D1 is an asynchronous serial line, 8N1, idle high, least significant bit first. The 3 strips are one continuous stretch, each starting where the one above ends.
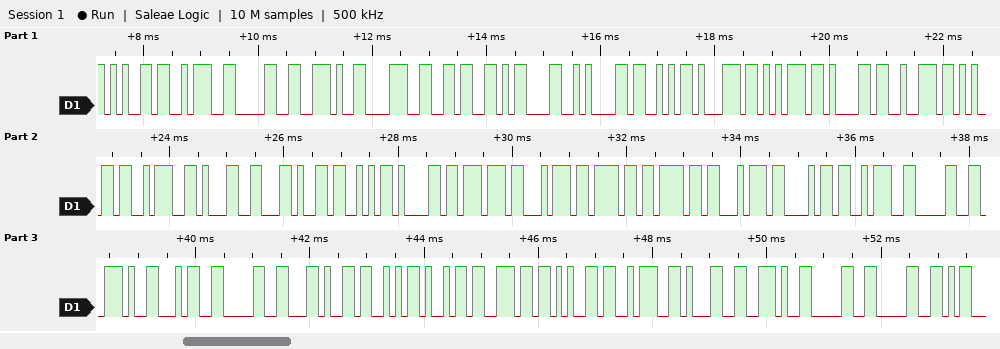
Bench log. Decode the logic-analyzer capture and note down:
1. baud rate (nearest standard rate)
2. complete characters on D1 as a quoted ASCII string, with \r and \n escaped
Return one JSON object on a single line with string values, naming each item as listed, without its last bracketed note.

{"baud rate": "9600 baud", "complete characters on D1 as a quoted ASCII string, with \\r and \\n escaped": "\"e:0.86\\r\\nSquare:1,Sawtooth:0.40,Sine:1.00\""}
